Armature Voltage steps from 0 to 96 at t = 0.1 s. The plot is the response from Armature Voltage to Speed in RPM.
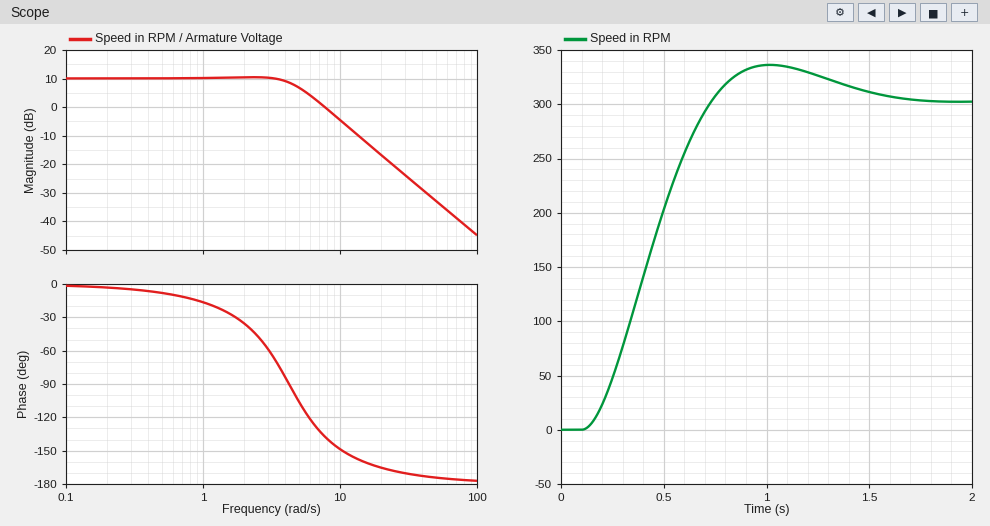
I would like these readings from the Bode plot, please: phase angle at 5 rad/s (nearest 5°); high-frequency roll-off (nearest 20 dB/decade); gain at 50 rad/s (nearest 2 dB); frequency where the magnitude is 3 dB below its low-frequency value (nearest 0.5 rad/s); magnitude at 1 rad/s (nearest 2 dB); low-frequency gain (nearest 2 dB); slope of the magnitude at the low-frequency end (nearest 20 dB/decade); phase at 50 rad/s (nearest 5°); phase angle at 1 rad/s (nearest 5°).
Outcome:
-105°
-40 dB/decade
-32 dB
5.0 rad/s
10 dB
10 dB
0 dB/decade
-175°
-15°
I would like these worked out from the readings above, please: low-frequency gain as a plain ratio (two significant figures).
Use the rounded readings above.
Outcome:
3.2
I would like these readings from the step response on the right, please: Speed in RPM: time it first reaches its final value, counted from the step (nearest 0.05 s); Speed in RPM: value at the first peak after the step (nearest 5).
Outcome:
0.65 s
335
